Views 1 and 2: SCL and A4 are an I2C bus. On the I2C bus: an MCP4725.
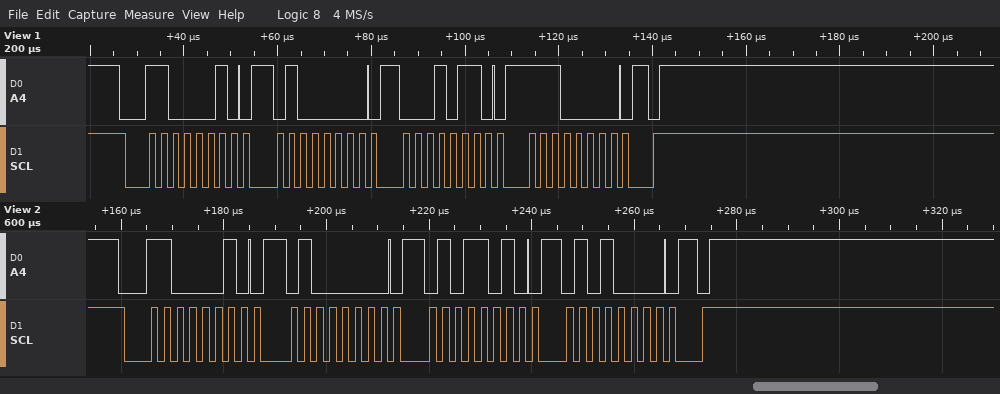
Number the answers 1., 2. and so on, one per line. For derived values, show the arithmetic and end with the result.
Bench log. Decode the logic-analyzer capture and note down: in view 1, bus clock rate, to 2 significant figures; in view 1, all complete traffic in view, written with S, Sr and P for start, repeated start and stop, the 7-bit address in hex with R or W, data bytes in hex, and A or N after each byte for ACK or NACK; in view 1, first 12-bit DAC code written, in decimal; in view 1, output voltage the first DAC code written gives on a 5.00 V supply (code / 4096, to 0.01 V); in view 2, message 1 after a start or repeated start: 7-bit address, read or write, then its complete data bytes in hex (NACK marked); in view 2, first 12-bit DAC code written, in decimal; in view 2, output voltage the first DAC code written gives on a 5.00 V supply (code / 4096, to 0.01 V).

1. 400 kHz
2. S 61W A 40 A 16 A E0 A P
3. 366
4. 366 / 4096 x 5.00 V = 0.45 V
5. 0x61 write: 40 5A 50
6. 1445
7. 1445 / 4096 x 5.00 V = 1.76 V
